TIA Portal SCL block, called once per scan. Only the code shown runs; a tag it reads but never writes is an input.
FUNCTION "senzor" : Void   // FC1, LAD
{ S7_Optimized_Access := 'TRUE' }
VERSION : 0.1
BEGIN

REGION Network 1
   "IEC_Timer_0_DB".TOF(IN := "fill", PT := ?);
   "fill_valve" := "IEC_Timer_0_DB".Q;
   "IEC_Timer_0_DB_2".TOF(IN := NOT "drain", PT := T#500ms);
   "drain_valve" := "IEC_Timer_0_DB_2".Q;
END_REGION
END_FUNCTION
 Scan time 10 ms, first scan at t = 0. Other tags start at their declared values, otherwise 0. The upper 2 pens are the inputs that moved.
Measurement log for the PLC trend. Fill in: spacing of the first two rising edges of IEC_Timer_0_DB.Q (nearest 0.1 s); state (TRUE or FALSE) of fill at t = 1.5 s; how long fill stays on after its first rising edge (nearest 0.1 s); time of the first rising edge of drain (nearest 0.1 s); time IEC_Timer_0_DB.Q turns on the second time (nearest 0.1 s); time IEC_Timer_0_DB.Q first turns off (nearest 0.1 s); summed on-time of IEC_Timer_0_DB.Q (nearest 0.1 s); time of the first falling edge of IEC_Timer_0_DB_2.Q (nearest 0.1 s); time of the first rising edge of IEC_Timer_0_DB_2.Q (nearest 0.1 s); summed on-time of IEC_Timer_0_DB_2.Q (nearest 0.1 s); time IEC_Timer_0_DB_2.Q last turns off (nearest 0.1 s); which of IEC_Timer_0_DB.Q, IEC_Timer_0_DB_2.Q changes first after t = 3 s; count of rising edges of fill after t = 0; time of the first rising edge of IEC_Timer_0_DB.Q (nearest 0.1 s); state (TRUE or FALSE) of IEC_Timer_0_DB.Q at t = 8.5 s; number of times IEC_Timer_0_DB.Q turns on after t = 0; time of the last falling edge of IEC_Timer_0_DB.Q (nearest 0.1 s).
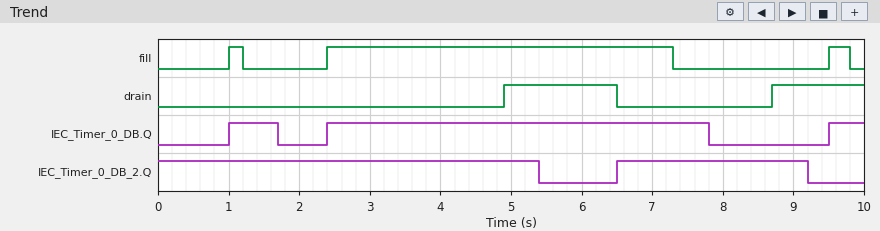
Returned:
1.4 s
FALSE
0.2 s
4.9 s
2.4 s
1.7 s
6.6 s
5.4 s
6.5 s
8.1 s
9.2 s
IEC_Timer_0_DB_2.Q
3
1.0 s
FALSE
3
7.8 s
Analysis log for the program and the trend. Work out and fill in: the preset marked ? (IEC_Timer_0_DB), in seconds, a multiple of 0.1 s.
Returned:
0.5 s
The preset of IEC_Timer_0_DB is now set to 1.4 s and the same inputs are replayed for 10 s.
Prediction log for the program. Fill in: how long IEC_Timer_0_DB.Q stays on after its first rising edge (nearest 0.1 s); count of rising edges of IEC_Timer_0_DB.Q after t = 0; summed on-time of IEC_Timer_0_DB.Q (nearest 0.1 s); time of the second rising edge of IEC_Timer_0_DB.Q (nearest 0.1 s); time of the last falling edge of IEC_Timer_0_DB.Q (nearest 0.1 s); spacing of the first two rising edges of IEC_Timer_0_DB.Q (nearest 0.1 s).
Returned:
7.7 s
2
8.2 s
9.5 s
8.7 s
8.5 s
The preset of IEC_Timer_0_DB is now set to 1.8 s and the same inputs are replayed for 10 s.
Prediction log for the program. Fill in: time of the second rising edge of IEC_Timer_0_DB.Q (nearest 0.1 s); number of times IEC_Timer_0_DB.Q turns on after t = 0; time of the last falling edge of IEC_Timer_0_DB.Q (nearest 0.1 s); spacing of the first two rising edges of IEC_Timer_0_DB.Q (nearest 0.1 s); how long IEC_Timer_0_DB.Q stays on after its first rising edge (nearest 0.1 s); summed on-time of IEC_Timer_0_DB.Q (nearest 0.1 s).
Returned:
9.5 s
2
9.1 s
8.5 s
8.1 s
8.6 s
